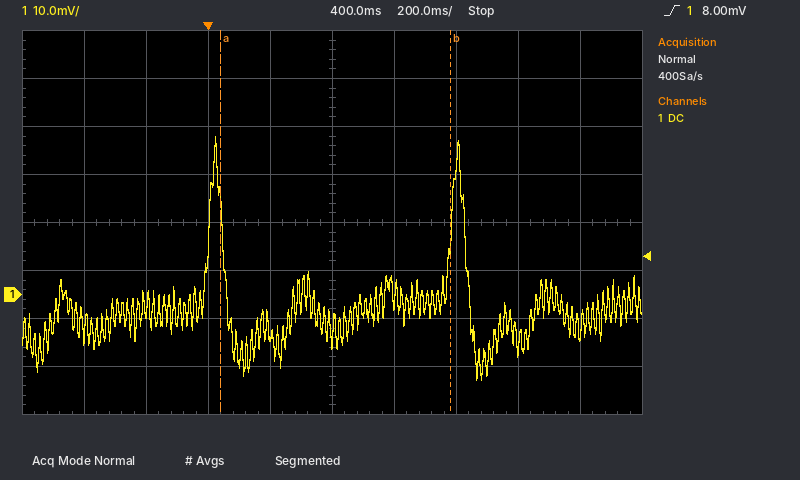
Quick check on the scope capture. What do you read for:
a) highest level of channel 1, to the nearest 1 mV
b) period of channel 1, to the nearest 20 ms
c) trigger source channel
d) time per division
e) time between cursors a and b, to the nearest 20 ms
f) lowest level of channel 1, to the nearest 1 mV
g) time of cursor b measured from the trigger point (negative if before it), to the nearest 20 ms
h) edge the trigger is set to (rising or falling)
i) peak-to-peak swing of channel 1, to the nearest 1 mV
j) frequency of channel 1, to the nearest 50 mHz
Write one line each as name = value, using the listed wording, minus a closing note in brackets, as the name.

highest level of channel 1, to the nearest 1 mV = 33 mV
period of channel 1, to the nearest 20 ms = 780 ms
trigger source channel = channel 1
time per division = 200 ms
time between cursors a and b, to the nearest 20 ms = 740 ms
lowest level of channel 1, to the nearest 1 mV = -18 mV
time of cursor b measured from the trigger point (negative if before it), to the nearest 20 ms = +780 ms
edge the trigger is set to = rising
peak-to-peak swing of channel 1, to the nearest 1 mV = 51 mV
frequency of channel 1, to the nearest 50 mHz = 1.30 Hz
